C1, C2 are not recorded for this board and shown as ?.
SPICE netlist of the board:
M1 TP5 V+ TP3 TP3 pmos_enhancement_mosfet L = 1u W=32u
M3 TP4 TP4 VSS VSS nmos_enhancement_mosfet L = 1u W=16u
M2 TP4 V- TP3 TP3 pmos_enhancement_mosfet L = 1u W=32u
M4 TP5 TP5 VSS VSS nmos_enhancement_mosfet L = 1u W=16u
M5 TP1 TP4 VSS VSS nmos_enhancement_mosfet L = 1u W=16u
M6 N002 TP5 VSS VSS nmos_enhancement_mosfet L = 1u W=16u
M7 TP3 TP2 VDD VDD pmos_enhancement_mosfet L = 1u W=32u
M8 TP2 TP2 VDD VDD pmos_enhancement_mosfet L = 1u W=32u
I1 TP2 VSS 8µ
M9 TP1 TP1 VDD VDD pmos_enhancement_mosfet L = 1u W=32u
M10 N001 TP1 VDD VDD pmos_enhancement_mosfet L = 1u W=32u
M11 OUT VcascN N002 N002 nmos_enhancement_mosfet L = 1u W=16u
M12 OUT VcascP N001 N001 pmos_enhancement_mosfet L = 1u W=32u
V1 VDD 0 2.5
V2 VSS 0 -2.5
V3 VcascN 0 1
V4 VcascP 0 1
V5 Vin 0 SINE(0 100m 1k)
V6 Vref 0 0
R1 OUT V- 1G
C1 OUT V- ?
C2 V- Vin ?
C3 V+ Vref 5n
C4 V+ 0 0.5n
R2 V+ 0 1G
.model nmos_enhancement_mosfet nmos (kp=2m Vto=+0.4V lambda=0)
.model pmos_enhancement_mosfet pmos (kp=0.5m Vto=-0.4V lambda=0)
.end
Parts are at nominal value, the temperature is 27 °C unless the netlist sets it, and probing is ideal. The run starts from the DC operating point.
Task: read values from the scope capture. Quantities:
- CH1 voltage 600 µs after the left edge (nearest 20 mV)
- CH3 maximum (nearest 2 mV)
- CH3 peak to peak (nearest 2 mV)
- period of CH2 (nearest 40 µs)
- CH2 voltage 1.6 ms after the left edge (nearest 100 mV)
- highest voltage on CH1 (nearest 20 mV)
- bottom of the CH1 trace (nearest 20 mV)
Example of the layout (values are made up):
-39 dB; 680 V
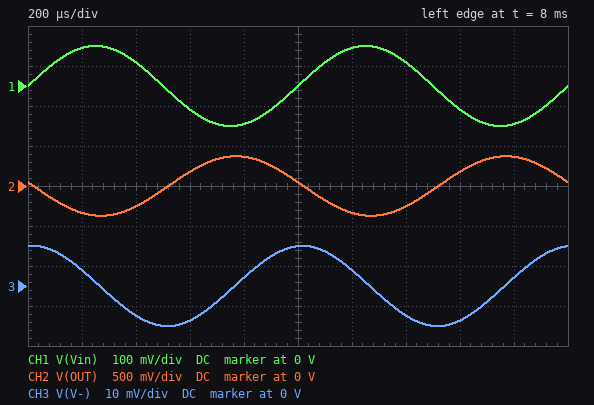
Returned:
-60 mV; 10 mV; 20 mV; 1.00 ms; 200 mV; 100 mV; -100 mV
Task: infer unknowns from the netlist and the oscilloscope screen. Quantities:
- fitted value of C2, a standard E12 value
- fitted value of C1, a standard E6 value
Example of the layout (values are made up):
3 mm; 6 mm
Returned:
5.6 nF; 1.5 nF
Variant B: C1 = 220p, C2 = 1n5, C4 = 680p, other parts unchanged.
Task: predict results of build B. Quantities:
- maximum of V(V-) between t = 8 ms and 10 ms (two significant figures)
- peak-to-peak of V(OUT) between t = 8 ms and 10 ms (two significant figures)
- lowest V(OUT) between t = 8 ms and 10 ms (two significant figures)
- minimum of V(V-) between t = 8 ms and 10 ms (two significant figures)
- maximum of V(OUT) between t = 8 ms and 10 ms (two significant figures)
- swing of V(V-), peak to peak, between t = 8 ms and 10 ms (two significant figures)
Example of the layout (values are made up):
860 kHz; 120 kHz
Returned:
2.6 mV; 1.4 V; -680 mV; -2.6 mV; 680 mV; 5.3 mV
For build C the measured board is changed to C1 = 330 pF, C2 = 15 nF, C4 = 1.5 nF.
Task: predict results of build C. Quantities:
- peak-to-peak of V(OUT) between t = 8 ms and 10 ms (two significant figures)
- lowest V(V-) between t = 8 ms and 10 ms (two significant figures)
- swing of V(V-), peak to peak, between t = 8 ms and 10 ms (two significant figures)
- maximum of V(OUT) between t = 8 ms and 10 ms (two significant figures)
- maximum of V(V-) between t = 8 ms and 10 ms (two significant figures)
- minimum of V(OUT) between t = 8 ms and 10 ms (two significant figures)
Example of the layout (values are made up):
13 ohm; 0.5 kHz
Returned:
5.0 V; -44 mV; 88 mV; 2.5 V; 44 mV; -2.5 V
